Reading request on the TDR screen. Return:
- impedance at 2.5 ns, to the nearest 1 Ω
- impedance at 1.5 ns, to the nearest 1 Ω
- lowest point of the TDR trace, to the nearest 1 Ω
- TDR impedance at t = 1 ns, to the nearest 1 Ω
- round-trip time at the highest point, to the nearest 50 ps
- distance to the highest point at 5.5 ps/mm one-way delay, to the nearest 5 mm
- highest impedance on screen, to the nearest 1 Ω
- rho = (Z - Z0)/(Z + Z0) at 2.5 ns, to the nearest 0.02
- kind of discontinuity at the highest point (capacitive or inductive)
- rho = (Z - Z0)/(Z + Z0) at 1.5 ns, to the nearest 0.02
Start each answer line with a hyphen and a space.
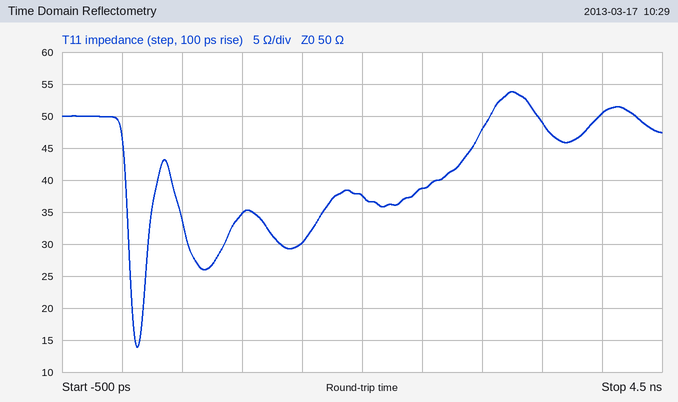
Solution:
- 39 Ω
- 30 Ω
- 14 Ω
- 35 Ω
- 3.25 ns
- 295 mm
- 54 Ω
- -0.12
- inductive
- -0.24
